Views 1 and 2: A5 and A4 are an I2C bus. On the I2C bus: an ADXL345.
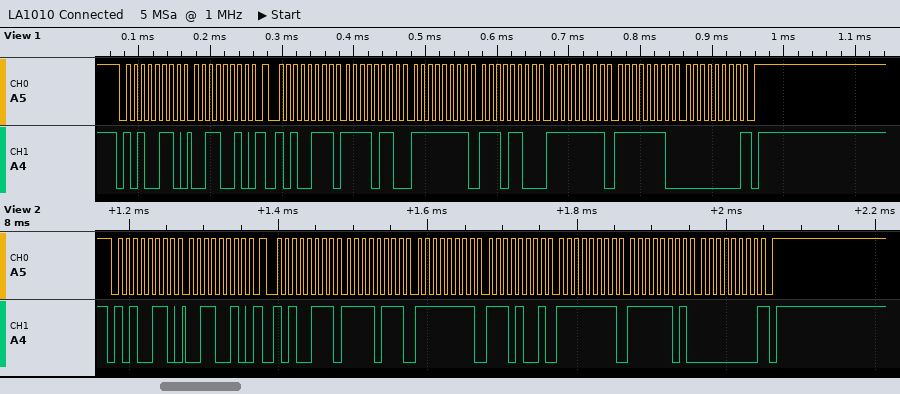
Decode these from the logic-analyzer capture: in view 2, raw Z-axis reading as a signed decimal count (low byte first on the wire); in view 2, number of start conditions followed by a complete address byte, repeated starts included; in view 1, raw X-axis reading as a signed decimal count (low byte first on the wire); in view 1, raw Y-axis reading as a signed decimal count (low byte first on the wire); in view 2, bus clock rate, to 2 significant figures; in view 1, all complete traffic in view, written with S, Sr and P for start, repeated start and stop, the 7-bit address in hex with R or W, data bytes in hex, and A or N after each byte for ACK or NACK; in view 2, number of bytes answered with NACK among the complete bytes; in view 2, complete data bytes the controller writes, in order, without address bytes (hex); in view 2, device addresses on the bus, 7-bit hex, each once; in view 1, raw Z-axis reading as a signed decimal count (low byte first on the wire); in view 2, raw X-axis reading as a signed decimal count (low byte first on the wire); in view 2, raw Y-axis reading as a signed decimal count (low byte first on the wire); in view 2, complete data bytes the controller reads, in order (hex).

253
2
-10
-20
100 kHz
S 53W A 32 A Sr 53R A F6 A FF A EC A FF A FE A 00 N P
1
32
0x53
254
-9
-23
F7 FF E9 FF FD 00
